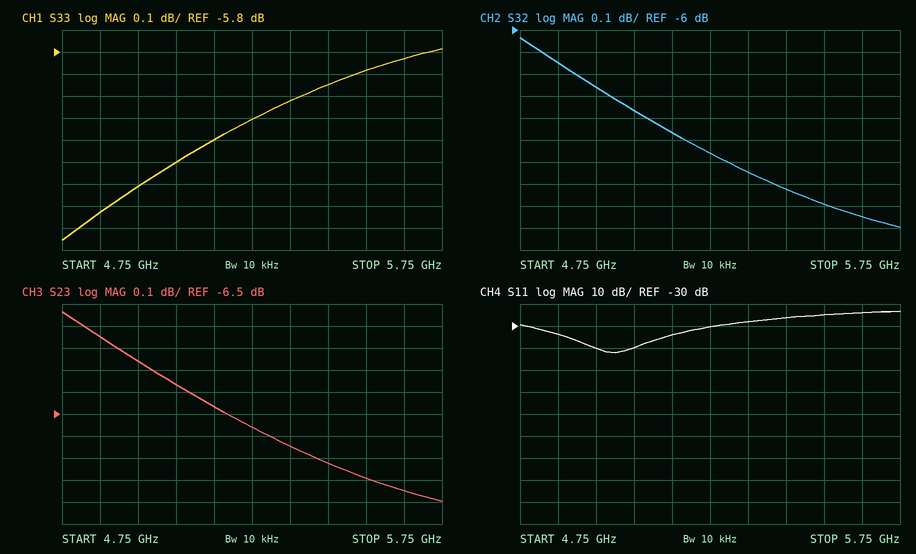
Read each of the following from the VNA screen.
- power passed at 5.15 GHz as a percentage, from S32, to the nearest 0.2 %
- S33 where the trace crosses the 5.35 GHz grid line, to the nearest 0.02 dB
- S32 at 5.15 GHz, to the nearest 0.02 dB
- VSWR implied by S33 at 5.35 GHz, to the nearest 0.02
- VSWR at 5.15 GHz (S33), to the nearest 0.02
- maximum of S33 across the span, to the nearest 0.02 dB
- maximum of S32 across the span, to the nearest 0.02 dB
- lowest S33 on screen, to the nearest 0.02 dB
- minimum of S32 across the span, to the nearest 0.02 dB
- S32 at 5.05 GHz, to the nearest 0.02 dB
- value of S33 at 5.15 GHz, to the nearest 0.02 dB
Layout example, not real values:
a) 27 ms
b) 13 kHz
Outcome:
a) 22.6 %
b) -6.02 dB
c) -6.46 dB
d) 3.00
e) 2.92
f) -5.78 dB
g) -6.04 dB
h) -6.66 dB
i) -6.90 dB
j) -6.36 dB
k) -6.20 dB
